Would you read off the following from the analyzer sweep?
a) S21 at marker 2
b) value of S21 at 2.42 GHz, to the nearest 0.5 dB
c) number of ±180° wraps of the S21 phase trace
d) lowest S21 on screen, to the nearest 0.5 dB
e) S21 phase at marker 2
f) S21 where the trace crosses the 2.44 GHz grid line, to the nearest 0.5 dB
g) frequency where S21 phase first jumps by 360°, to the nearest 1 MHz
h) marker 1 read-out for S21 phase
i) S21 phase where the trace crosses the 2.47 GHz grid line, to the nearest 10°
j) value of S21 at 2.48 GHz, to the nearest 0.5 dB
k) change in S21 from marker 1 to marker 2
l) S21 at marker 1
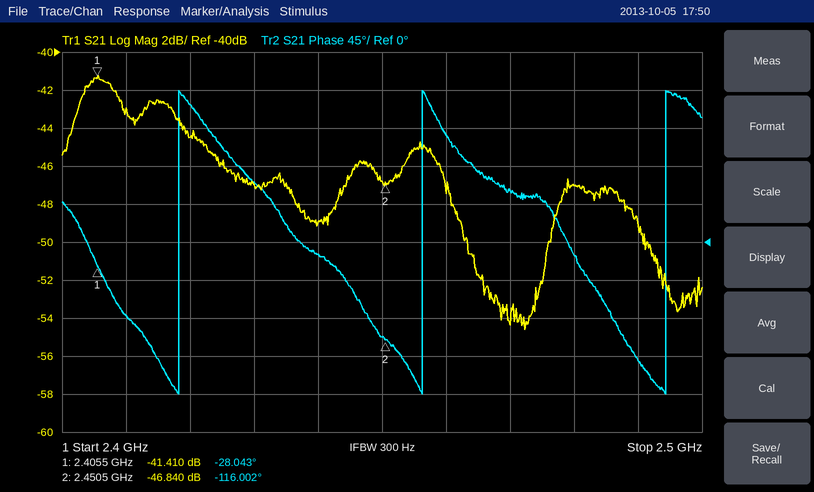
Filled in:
-46.840 dB
-44.5 dB
3
-54.5 dB
-116.002°
-49.0 dB
2.418 GHz
-28.043°
60°
-47.0 dB
-5.430 dB
-41.410 dB
